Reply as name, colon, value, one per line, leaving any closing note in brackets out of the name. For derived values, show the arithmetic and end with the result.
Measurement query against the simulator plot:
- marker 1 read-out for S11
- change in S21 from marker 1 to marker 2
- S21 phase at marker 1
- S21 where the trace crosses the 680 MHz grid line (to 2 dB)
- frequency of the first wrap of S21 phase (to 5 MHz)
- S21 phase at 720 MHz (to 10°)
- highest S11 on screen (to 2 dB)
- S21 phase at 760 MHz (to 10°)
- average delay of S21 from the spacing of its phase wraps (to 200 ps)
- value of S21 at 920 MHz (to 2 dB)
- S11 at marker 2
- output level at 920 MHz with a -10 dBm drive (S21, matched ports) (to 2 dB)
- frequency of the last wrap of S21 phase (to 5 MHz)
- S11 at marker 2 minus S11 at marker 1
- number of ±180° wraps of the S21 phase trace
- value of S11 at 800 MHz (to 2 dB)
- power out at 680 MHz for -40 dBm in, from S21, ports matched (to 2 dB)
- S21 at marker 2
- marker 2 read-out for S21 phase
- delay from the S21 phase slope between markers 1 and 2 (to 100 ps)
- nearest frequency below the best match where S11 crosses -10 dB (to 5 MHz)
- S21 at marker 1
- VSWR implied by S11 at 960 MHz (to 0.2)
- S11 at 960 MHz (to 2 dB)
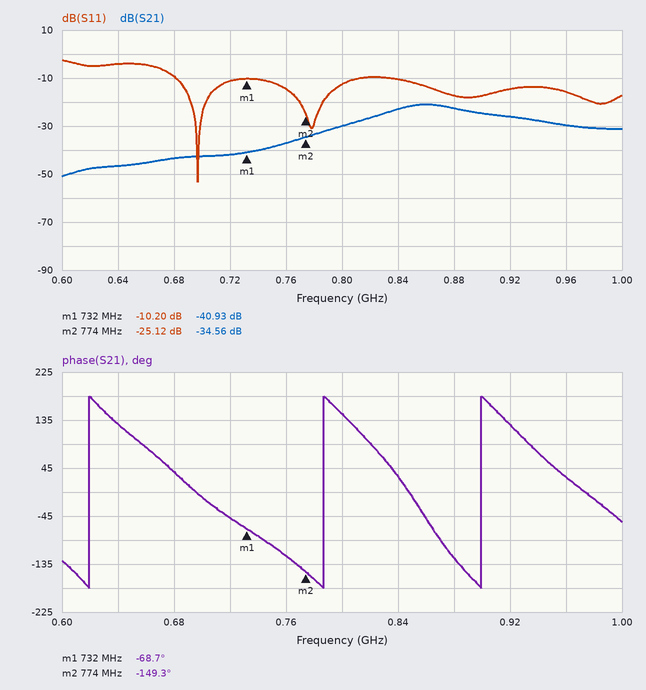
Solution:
marker 1 read-out for S11: -10.20 dB
change in S21 from marker 1 to marker 2: -34.56 − (-40.93) = 6.37 dB
S21 phase at marker 1: -68.7°
S21 where the trace crosses the 680 MHz grid line: -44 dB
frequency of the first wrap of S21 phase: 620 MHz
S21 phase at 720 MHz: -50°
highest S11 on screen: -2 dB
S21 phase at 760 MHz: -120°
average delay of S21 from the spacing of its phase wraps: 2 cycles / (900 MHz − 620 MHz) ≈ 7.14 ns, so 7.2 ns to the nearest 200 ps
value of S21 at 920 MHz: -26 dB
S11 at marker 2: -25.12 dB
output level at 920 MHz with a -10 dBm drive (S21, matched ports): -10 dBm + (-26 dB) = -36 dBm
frequency of the last wrap of S21 phase: 900 MHz
S11 at marker 2 minus S11 at marker 1: -25.12 − (-10.2) = -14.92 dB
number of ±180° wraps of the S21 phase trace: 3
value of S11 at 800 MHz: -12 dB
power out at 680 MHz for -40 dBm in, from S21, ports matched: -40 dBm + (-44 dB) = -84 dBm
S21 at marker 2: -34.56 dB
marker 2 read-out for S21 phase: -149.3°
delay from the S21 phase slope between markers 1 and 2: −(-149.3° − (-68.7°))/(360° × 42 MHz) ≈ 5.3 ns
nearest frequency below the best match where S11 crosses -10 dB: 680 MHz
S21 at marker 1: -40.93 dB
VSWR implied by S11 at 960 MHz: |Γ| = 10^(-16/20) = 0.1585; VSWR = (1 + 0.1585)/(1 − 0.1585) ≈ 1.4
S11 at 960 MHz: -16 dB
